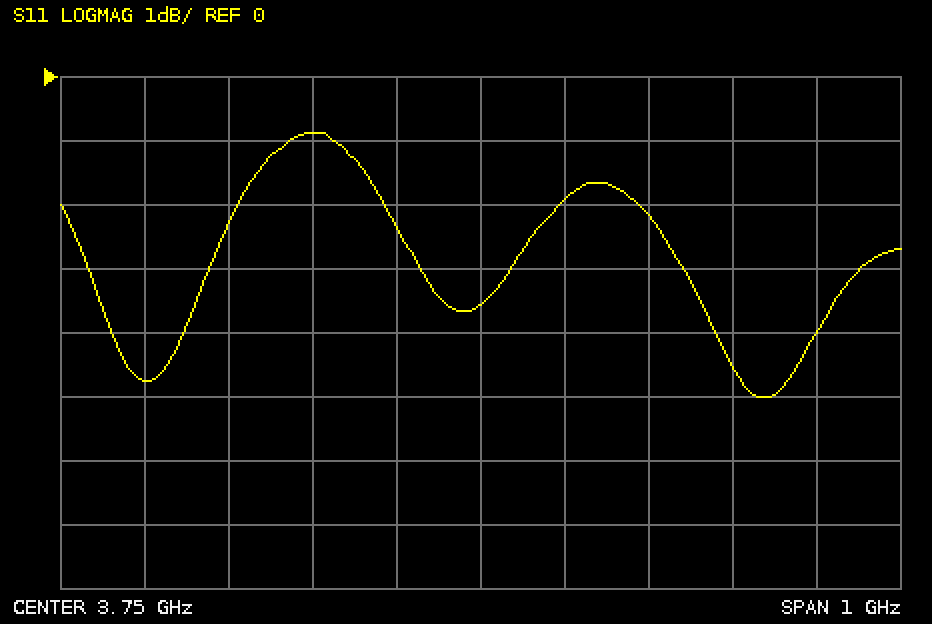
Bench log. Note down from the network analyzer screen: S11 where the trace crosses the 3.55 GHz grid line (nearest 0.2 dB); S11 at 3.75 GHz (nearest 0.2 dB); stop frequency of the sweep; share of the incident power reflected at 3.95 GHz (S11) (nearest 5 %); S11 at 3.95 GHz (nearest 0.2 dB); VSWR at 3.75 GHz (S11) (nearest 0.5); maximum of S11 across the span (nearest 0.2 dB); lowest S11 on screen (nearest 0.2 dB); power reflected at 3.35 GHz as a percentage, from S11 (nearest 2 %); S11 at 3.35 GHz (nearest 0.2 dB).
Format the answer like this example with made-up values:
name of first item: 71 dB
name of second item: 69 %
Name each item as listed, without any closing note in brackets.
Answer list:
S11 where the trace crosses the 3.55 GHz grid line: -0.8 dB
S11 at 3.75 GHz: -3.6 dB
stop frequency of the sweep: 4.25 GHz
share of the incident power reflected at 3.95 GHz (S11): 60 %
S11 at 3.95 GHz: -2.2 dB
VSWR at 3.75 GHz (S11): 5.0
maximum of S11 across the span: -0.8 dB
lowest S11 on screen: -5.0 dB
power reflected at 3.35 GHz as a percentage, from S11: 34 %
S11 at 3.35 GHz: -4.8 dB
